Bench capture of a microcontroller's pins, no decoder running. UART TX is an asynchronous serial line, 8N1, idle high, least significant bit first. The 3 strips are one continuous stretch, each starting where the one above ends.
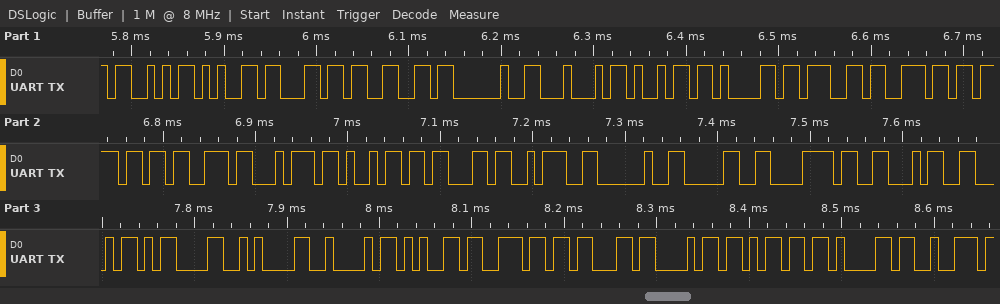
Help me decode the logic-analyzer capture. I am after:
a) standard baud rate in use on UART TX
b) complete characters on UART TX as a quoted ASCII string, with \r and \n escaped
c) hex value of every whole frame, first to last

115200 baud
"Self Diagnostic: 0xFF\r\nBenchmar"
53 65 6C 66 20 44 69 61 67 6E 6F 73 74 69 63 3A 20 30 78 46 46 0D 0A 42 65 6E 63 68 6D 61 72
